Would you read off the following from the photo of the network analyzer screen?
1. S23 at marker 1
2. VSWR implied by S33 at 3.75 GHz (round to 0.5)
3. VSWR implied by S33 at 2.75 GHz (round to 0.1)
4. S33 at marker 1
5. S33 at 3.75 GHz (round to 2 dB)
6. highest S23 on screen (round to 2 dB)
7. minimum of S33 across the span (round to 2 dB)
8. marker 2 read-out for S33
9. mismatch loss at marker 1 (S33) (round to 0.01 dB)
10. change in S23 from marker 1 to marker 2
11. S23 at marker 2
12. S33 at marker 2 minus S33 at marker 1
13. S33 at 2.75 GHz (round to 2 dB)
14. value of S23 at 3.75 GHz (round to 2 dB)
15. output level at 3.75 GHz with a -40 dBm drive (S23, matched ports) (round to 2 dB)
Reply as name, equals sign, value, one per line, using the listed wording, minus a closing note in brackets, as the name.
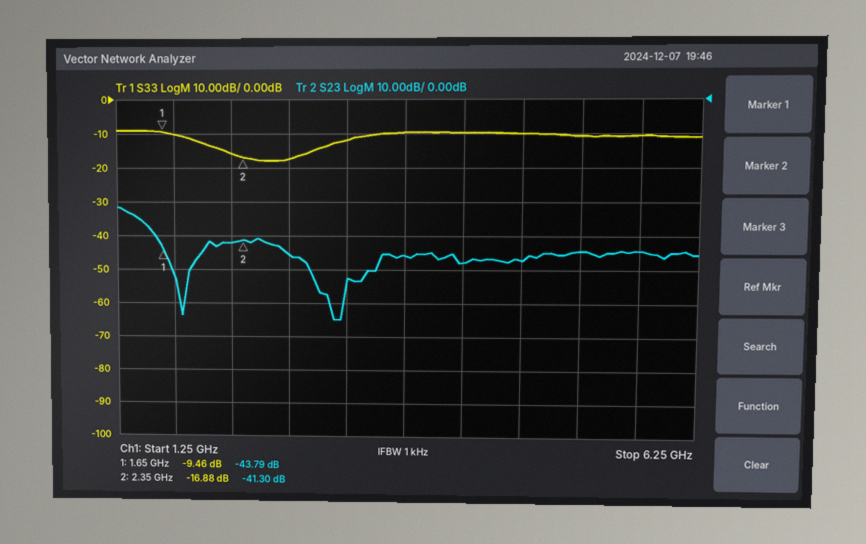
S23 at marker 1 = -43.79 dB
VSWR implied by S33 at 3.75 GHz = 2.0
VSWR implied by S33 at 2.75 GHz = 1.3
S33 at marker 1 = -9.46 dB
S33 at 3.75 GHz = -10 dB
highest S23 on screen = -32 dB
minimum of S33 across the span = -18 dB
marker 2 read-out for S33 = -16.88 dB
mismatch loss at marker 1 (S33) = 0.52 dB
change in S23 from marker 1 to marker 2 = 2.49 dB
S23 at marker 2 = -41.30 dB
S33 at marker 2 minus S33 at marker 1 = -7.42 dB
S33 at 2.75 GHz = -18 dB
value of S23 at 3.75 GHz = -46 dB
output level at 3.75 GHz with a -40 dBm drive (S23, matched ports) = -86 dBm
